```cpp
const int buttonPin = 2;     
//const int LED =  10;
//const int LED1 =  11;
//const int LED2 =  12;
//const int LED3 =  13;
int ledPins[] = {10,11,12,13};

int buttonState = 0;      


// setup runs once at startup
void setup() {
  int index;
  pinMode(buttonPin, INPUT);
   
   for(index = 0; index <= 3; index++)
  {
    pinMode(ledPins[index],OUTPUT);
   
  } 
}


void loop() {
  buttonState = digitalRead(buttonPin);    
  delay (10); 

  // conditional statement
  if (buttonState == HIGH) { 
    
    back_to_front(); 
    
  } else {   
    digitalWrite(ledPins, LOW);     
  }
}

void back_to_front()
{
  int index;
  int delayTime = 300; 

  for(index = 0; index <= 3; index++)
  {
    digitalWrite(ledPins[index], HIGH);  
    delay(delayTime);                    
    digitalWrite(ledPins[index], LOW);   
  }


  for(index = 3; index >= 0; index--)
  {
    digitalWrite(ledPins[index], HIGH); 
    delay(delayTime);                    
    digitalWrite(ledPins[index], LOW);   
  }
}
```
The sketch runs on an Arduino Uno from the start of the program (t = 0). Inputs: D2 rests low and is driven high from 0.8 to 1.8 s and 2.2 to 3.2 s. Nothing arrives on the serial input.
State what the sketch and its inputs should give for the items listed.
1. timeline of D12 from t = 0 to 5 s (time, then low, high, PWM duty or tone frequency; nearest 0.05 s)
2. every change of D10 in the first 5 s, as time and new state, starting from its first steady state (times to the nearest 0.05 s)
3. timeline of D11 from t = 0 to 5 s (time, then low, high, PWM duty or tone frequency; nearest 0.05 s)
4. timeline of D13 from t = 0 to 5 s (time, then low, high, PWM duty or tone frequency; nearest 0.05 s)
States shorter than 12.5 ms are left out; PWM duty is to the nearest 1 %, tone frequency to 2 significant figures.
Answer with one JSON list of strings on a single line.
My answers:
["0 s low; 1.4 s high; 1.7 s low; 2.3 s high; 2.6 s low", "0 s low; 0.8 s high; 1.1 s low; 2.9 s high; 3.2 s low", "0 s low; 1.1 s high; 1.4 s low; 2.6 s high; 2.9 s low", "0 s low; 1.7 s high; 2.3 s low"]
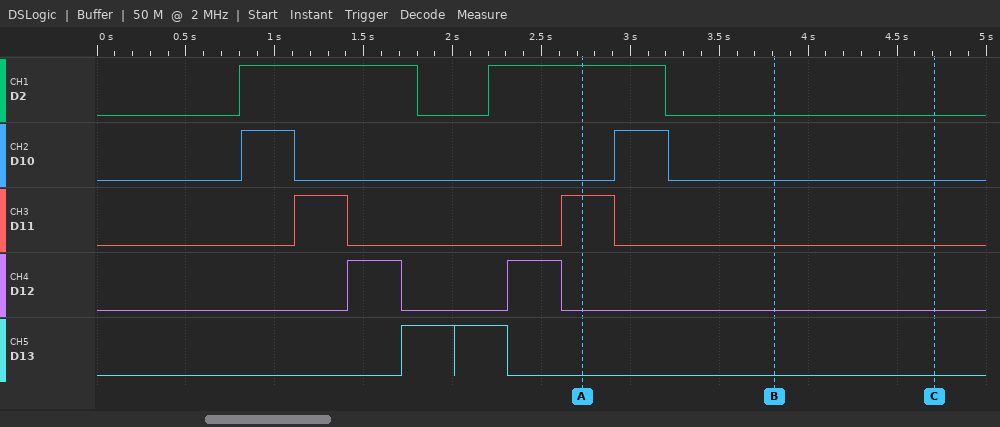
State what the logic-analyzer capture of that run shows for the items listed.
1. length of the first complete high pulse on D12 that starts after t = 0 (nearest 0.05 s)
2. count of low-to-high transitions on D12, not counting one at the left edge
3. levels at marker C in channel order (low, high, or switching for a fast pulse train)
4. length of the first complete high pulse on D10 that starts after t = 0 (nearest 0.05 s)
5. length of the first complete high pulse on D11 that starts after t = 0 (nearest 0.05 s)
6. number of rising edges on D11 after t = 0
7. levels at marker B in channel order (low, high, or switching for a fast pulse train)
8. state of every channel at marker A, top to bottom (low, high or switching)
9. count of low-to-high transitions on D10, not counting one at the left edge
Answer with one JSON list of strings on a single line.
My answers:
["0.30 s", "2", "D2 low, D10 low, D11 low, D12 low, D13 low", "0.30 s", "0.30 s", "2", "D2 low, D10 low, D11 low, D12 low, D13 low", "D2 high, D10 low, D11 high, D12 low, D13 low", "2"]
